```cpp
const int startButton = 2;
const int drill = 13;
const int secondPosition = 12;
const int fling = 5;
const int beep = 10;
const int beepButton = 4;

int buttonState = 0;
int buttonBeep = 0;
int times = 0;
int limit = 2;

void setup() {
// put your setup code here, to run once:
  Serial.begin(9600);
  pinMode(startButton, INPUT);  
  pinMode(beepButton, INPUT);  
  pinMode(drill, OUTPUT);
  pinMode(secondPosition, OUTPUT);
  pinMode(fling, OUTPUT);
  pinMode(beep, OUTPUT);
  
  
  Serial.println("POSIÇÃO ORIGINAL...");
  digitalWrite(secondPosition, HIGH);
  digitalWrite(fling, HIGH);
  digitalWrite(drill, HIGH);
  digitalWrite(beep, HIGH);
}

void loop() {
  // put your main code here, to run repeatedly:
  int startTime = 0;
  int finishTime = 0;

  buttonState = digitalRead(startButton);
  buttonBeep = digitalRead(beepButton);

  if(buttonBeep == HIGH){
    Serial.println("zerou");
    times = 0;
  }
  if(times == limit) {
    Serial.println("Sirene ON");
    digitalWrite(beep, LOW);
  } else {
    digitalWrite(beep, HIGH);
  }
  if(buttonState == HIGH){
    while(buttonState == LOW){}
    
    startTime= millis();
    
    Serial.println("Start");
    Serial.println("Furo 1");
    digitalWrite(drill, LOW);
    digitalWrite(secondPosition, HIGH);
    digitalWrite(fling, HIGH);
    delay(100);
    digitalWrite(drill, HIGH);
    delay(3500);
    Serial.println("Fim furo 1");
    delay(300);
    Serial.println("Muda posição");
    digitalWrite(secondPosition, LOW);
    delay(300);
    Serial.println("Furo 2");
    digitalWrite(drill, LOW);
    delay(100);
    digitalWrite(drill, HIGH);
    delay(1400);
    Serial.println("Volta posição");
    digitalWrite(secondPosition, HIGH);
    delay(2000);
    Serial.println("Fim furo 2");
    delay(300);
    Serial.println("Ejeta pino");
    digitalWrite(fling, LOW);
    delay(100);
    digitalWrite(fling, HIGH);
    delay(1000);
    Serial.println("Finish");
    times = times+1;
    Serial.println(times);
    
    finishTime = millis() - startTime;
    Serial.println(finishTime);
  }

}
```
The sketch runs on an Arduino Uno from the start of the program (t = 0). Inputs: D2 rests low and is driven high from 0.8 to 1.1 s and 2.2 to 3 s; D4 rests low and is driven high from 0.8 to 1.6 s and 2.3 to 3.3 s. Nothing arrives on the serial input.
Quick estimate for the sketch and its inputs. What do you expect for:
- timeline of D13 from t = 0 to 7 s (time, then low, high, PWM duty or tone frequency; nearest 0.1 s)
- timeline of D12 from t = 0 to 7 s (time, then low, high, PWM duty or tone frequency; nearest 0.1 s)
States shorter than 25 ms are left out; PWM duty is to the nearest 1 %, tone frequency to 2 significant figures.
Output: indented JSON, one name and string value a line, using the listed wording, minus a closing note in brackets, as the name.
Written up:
{
  "timeline of D13 from t = 0 to 7 s": "0 s high; 0.8 s low; 0.9 s high; 5 s low; 5.1 s high",
  "timeline of D12 from t = 0 to 7 s": "0 s high; 4.7 s low; 6.5 s high"
}
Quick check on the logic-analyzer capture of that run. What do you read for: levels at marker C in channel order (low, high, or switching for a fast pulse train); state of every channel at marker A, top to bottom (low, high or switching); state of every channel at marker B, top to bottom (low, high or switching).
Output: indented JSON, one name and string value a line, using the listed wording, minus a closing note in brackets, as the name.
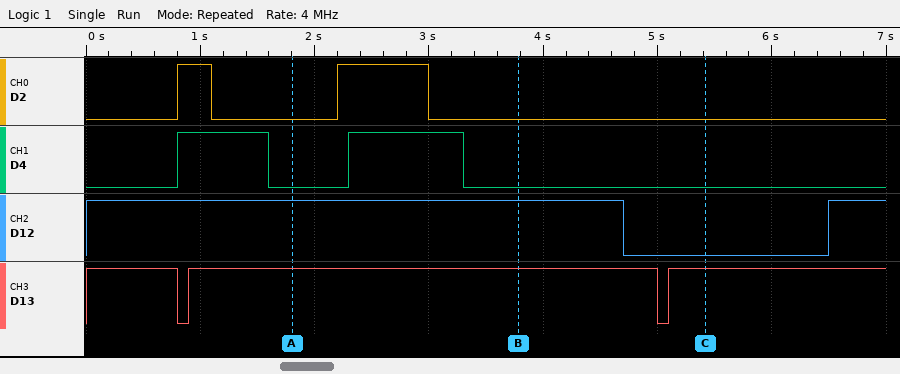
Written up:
{
  "levels at marker C in channel order": "D2 low, D4 low, D12 low, D13 high",
  "state of every channel at marker A, top to bottom": "D2 low, D4 low, D12 high, D13 high",
  "state of every channel at marker B, top to bottom": "D2 low, D4 low, D12 high, D13 high"
}
